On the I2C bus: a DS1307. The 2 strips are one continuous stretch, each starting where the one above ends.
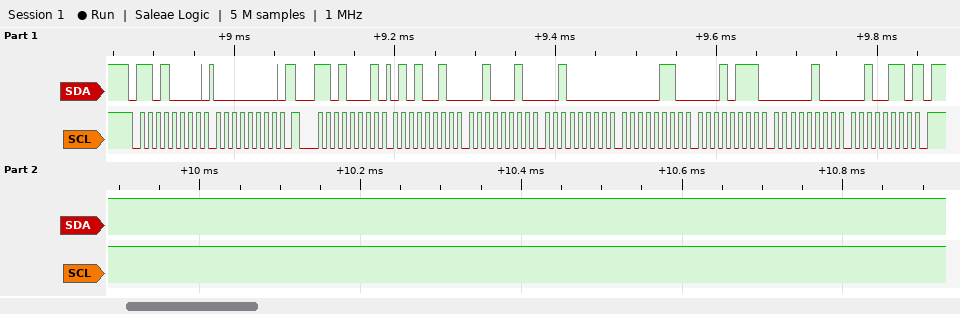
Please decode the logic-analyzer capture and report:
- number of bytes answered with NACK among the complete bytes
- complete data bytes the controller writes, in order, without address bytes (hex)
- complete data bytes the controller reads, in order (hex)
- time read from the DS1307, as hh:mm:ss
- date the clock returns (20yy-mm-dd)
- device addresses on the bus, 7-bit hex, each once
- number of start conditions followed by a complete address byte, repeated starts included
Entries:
1
00
52 22 20 06 17 04 26
20:22:52
2026-04-17
0x68
2
